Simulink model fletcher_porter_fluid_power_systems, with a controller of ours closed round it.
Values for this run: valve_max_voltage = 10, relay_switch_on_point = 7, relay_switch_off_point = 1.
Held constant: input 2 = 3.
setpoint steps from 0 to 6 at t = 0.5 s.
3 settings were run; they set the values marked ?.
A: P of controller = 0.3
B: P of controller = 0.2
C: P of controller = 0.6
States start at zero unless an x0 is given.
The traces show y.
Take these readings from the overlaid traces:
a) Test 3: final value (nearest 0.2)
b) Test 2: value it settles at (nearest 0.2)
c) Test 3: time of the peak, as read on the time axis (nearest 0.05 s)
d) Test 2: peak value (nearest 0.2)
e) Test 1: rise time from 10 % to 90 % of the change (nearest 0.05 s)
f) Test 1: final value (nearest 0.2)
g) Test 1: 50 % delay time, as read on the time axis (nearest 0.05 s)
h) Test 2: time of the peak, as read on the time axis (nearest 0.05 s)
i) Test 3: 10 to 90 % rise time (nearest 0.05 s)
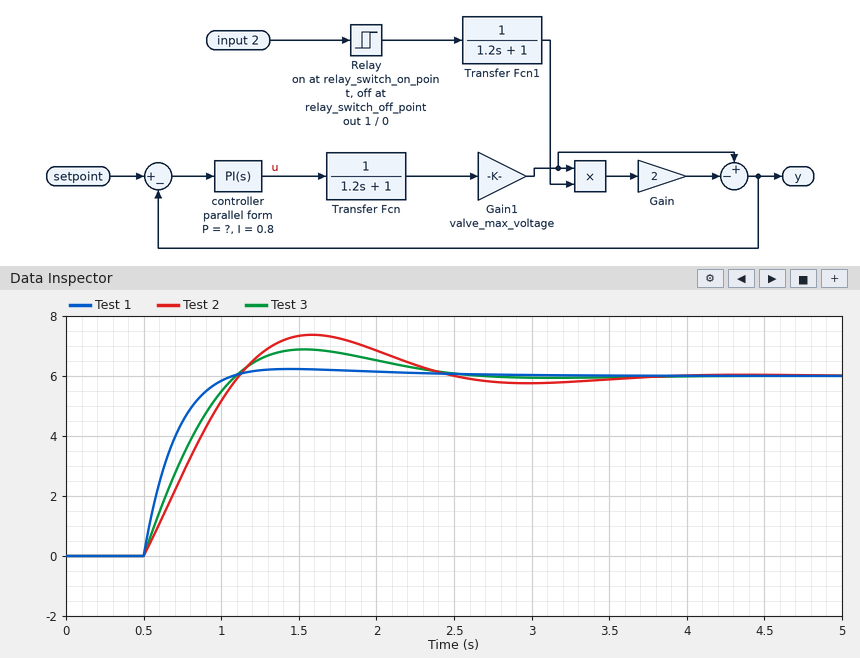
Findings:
6.0
6.0
1.55 s
7.4
0.35 s
6.0
0.65 s
1.60 s
0.45 s
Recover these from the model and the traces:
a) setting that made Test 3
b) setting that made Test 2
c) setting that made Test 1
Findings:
A
B
C
